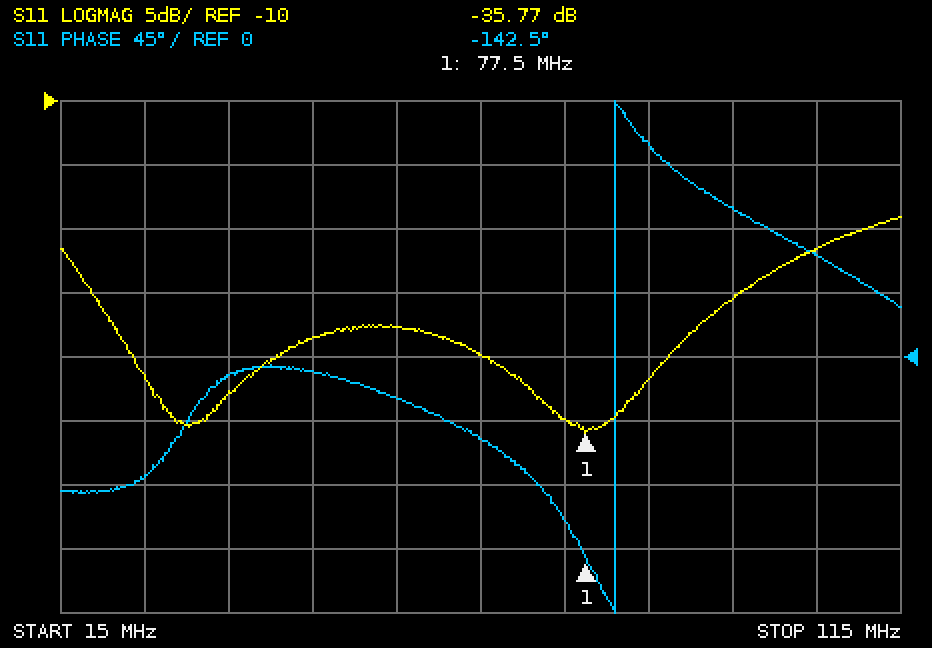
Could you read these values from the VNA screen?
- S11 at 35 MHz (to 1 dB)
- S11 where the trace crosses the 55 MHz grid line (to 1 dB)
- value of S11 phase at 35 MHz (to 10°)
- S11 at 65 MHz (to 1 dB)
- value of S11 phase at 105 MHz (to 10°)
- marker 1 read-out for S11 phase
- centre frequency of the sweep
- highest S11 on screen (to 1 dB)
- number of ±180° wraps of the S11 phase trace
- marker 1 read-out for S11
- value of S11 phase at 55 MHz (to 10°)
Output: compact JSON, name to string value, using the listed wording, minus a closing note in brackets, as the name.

{"S11 at 35 MHz": "-33 dB", "S11 where the trace crosses the 55 MHz grid line": "-28 dB", "value of S11 phase at 35 MHz": "-10°", "S11 at 65 MHz": "-30 dB", "value of S11 phase at 105 MHz": "70°", "marker 1 read-out for S11 phase": "-142.5°", "centre frequency of the sweep": "65 MHz", "highest S11 on screen": "-19 dB", "number of ±180° wraps of the S11 phase trace": "1", "marker 1 read-out for S11": "-35.77 dB", "value of S11 phase at 55 MHz": "-30°"}
